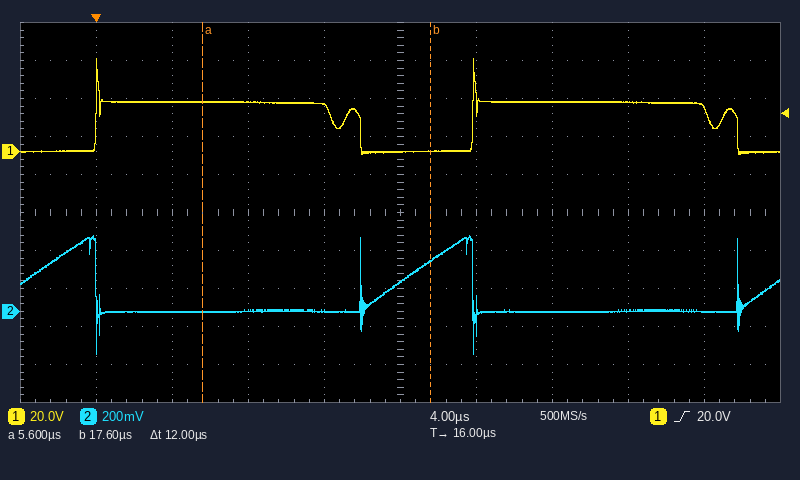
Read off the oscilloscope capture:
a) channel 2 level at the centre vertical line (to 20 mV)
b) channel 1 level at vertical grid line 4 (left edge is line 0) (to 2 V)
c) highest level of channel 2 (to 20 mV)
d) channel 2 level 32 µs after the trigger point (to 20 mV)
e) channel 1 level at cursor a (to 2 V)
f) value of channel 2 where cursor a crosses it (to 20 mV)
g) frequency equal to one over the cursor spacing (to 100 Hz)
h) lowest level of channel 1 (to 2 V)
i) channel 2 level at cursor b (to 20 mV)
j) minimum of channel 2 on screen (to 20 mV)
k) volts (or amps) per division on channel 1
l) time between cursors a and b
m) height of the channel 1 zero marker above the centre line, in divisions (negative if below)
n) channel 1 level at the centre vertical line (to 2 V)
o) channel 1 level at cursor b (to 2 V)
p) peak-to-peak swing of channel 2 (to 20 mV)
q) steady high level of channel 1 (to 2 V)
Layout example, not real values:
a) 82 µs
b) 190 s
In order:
a) 160 mV
b) 24 V
c) 400 mV
d) 0 mV
e) 26 V
f) 0 mV
g) 83.3 kHz
h) -2 V
i) 260 mV
j) -220 mV
k) 20 V
l) 12 µs
m) +1.6 div
n) 0 V
o) 0 V
p) 620 mV
q) 26 V
